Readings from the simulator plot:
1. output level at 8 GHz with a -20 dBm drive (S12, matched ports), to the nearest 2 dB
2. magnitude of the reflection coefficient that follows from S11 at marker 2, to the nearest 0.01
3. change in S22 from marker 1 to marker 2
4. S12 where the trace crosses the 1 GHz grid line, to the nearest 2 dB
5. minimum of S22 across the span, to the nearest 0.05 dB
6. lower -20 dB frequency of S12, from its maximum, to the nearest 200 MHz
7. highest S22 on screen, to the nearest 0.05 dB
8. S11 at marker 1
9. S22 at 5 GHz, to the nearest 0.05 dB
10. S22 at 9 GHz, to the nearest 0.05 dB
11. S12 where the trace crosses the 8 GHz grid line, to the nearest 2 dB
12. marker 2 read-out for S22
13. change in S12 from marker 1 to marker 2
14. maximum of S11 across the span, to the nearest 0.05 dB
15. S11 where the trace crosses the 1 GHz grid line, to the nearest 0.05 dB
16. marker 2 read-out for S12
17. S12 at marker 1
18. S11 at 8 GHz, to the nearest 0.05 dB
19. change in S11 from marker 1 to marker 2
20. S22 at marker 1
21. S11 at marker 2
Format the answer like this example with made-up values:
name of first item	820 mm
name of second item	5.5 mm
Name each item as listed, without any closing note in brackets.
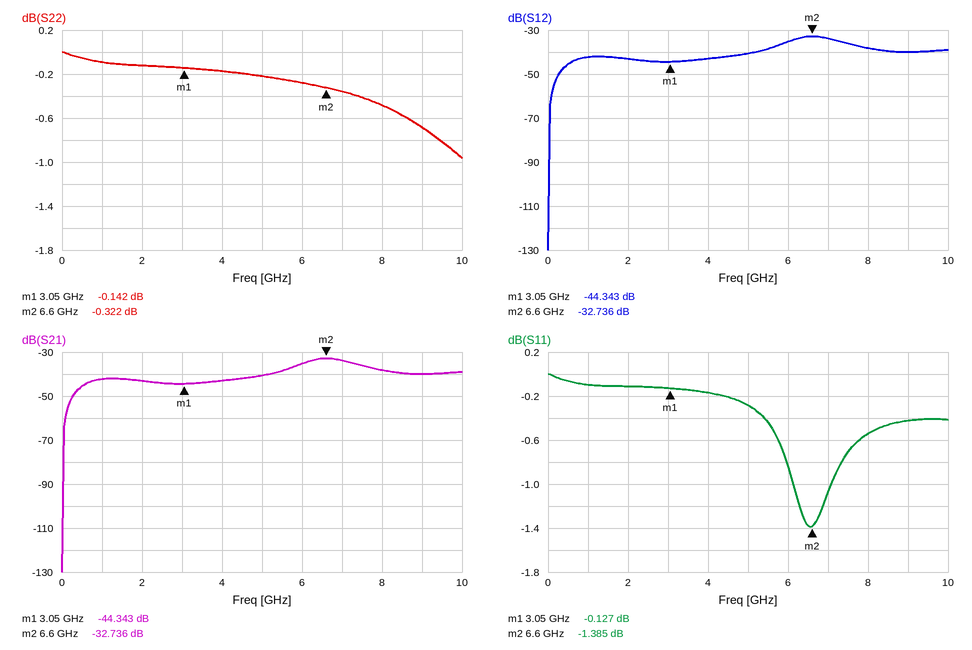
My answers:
output level at 8 GHz with a -20 dBm drive (S12, matched ports), to the nearest 2 dB	-58 dBm
magnitude of the reflection coefficient that follows from S11 at marker 2, to the nearest 0.01	0.85
change in S22 from marker 1 to marker 2	-0.180 dB
S12 where the trace crosses the 1 GHz grid line, to the nearest 2 dB	-42 dB
minimum of S22 across the span, to the nearest 0.05 dB	-0.95 dB
lower -20 dB frequency of S12, from its maximum, to the nearest 200 MHz	200 MHz
highest S22 on screen, to the nearest 0.05 dB	0.00 dB
S11 at marker 1	-0.127 dB
S22 at 5 GHz, to the nearest 0.05 dB	-0.20 dB
S22 at 9 GHz, to the nearest 0.05 dB	-0.70 dB
S12 where the trace crosses the 8 GHz grid line, to the nearest 2 dB	-38 dB
marker 2 read-out for S22	-0.322 dB
change in S12 from marker 1 to marker 2	11.607 dB
maximum of S11 across the span, to the nearest 0.05 dB	0.00 dB
S11 where the trace crosses the 1 GHz grid line, to the nearest 0.05 dB	-0.10 dB
marker 2 read-out for S12	-32.736 dB
S12 at marker 1	-44.343 dB
S11 at 8 GHz, to the nearest 0.05 dB	-0.55 dB
change in S11 from marker 1 to marker 2	-1.258 dB
S22 at marker 1	-0.142 dB
S11 at marker 2	-1.385 dB
